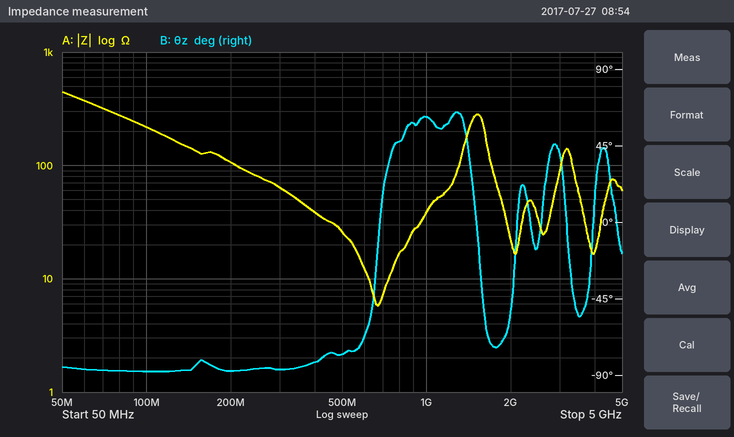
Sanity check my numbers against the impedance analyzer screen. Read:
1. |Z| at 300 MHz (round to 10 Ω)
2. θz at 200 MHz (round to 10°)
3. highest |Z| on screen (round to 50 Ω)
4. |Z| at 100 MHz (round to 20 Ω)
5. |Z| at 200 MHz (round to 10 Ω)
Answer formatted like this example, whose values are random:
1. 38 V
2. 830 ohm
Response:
1. 60 Ω
2. -90°
3. 450 Ω
4. 220 Ω
5. 110 Ω
